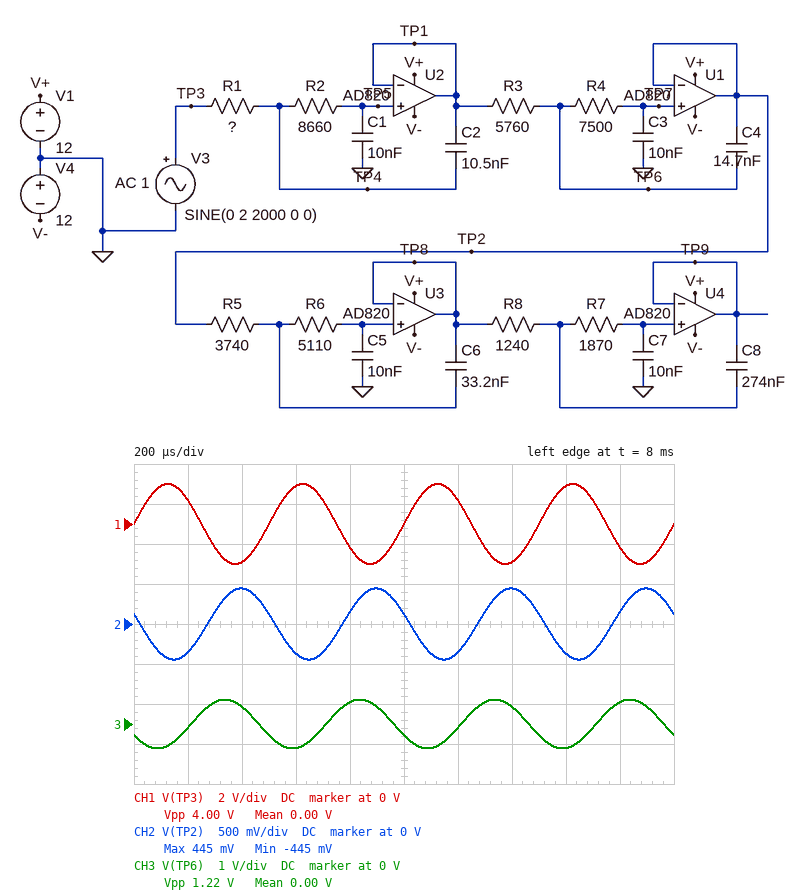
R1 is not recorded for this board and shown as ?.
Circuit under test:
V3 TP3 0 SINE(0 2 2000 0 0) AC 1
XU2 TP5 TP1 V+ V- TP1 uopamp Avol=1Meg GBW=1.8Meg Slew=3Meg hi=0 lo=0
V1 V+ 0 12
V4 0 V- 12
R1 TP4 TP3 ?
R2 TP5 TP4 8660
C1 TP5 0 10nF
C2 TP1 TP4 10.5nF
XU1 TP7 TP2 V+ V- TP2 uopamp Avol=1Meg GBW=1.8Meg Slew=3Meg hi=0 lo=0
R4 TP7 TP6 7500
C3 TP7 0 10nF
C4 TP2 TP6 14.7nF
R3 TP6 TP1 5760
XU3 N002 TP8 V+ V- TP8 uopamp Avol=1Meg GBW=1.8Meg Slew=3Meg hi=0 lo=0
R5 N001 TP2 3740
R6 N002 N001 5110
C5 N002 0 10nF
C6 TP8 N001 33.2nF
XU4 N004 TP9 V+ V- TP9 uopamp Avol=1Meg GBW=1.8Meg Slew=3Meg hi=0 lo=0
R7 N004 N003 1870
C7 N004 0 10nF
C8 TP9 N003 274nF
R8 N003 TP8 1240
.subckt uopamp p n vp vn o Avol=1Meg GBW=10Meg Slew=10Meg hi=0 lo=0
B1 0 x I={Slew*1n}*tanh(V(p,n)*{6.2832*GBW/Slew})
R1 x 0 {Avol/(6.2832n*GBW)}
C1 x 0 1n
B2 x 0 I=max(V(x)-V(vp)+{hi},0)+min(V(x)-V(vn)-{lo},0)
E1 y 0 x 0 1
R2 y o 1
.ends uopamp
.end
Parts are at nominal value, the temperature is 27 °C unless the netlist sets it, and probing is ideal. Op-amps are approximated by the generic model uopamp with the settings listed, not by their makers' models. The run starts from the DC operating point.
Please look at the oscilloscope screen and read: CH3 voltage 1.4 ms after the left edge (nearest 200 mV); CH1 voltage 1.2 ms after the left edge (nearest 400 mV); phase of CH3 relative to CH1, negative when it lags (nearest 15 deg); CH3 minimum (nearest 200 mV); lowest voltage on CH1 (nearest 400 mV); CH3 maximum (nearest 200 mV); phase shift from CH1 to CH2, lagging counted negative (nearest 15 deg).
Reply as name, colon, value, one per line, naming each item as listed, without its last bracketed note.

CH3 voltage 1.4 ms after the left edge: 400 mV
CH1 voltage 1.2 ms after the left edge: 1.2 V
phase of CH3 relative to CH1, negative when it lags: -150 deg
CH3 minimum: -600 mV
lowest voltage on CH1: -2.0 V
CH3 maximum: 600 mV
phase shift from CH1 to CH2, lagging counted negative: 165 deg
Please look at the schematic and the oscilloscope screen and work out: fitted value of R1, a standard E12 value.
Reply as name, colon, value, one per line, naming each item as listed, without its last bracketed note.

fitted value of R1, a standard E12 value: 12 kΩ
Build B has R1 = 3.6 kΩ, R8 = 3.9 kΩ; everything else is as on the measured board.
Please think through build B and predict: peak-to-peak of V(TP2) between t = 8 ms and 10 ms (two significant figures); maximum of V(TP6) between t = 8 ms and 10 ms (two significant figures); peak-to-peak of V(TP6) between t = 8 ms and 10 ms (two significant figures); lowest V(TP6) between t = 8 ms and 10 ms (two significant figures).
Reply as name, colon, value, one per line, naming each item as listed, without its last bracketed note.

peak-to-peak of V(TP2) between t = 8 ms and 10 ms: 1.5 V
maximum of V(TP6) between t = 8 ms and 10 ms: 1.0 V
peak-to-peak of V(TP6) between t = 8 ms and 10 ms: 2.0 V
lowest V(TP6) between t = 8 ms and 10 ms: -1.0 V
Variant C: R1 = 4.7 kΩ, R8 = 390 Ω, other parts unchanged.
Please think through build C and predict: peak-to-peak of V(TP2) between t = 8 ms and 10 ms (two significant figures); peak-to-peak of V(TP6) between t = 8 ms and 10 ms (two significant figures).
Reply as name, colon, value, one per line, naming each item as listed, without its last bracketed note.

peak-to-peak of V(TP2) between t = 8 ms and 10 ms: 1.4 V
peak-to-peak of V(TP6) between t = 8 ms and 10 ms: 1.9 V
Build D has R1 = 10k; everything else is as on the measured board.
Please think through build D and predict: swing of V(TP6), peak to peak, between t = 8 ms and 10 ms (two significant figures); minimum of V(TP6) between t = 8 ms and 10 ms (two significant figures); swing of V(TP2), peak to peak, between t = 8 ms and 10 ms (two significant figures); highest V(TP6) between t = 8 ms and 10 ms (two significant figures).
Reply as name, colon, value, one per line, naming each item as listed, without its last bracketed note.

swing of V(TP6), peak to peak, between t = 8 ms and 10 ms: 1.4 V
minimum of V(TP6) between t = 8 ms and 10 ms: -690 mV
swing of V(TP2), peak to peak, between t = 8 ms and 10 ms: 1.0 V
highest V(TP6) between t = 8 ms and 10 ms: 690 mV
